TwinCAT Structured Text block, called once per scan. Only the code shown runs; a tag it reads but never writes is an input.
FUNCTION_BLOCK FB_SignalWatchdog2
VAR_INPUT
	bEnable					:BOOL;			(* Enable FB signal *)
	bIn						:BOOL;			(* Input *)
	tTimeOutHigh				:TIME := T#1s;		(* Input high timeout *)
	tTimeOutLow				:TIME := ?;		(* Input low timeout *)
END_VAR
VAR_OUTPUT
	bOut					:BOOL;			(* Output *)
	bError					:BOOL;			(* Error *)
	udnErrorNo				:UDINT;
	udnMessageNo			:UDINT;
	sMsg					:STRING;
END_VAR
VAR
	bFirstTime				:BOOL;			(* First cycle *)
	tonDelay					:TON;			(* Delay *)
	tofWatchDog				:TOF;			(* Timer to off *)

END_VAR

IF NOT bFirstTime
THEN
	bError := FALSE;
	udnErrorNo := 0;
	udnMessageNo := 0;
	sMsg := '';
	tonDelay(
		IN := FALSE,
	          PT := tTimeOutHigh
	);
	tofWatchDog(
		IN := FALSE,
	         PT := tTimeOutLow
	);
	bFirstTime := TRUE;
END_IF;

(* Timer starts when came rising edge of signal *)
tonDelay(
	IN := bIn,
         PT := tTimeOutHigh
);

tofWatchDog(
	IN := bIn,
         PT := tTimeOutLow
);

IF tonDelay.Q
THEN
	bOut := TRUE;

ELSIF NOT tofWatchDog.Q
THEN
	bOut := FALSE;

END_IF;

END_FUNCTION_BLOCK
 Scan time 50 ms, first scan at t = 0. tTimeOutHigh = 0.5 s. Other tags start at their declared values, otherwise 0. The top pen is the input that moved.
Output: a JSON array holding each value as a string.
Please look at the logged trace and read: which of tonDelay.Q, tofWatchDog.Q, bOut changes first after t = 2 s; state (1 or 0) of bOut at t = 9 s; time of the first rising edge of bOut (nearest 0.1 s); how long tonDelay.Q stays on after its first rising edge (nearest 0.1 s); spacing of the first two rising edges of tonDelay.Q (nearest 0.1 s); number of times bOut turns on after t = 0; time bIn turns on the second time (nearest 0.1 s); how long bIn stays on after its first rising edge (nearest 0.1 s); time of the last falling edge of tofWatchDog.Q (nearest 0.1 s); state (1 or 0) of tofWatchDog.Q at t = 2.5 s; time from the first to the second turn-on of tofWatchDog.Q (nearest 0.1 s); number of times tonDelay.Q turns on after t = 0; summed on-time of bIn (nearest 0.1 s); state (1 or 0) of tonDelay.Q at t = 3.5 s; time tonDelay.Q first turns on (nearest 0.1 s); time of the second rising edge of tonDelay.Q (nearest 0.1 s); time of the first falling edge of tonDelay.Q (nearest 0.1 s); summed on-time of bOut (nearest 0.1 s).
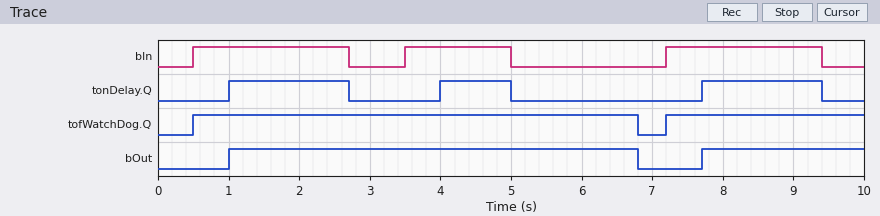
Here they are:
["tonDelay.Q", "1", "1.0 s", "1.7 s", "3.0 s", "2", "3.5 s", "2.2 s", "6.8 s", "1", "6.7 s", "3", "5.9 s", "0", "1.0 s", "4.0 s", "2.7 s", "8.1 s"]
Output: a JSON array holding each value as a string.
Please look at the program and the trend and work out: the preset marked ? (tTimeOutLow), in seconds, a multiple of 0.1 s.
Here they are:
["1.8 s"]
